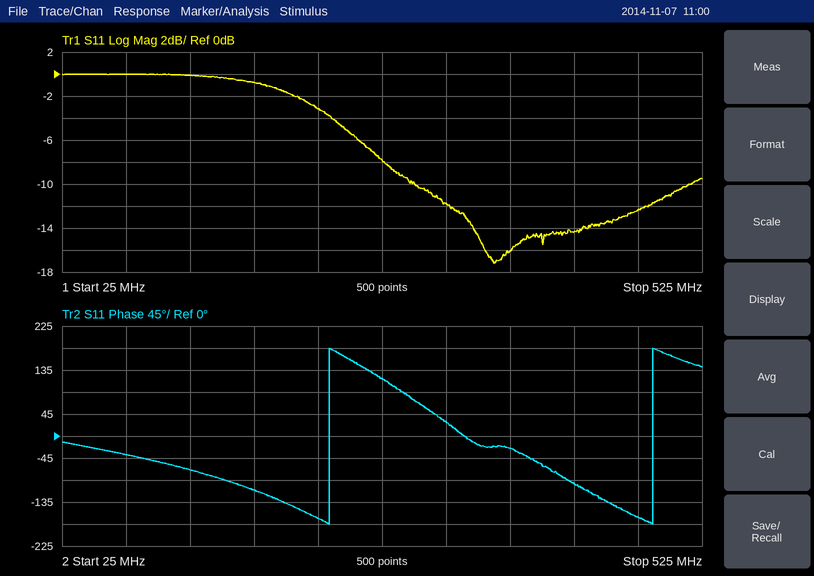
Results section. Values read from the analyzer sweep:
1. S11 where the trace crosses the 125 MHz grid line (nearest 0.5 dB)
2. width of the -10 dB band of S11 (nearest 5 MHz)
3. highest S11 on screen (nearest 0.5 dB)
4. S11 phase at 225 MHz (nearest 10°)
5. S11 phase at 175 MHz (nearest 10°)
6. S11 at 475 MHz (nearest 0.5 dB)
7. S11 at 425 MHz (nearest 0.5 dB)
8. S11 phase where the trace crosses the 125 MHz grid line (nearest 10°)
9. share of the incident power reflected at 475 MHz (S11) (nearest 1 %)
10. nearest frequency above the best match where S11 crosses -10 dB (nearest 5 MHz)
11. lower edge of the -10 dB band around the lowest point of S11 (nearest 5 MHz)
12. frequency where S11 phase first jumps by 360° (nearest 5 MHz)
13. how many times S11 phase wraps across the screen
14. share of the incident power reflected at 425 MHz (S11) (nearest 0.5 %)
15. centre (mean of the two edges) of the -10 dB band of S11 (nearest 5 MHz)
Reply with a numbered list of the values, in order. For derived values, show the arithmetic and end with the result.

1. 0.0 dB
2. 515 MHz − 300 MHz = 215 MHz
3. 0.0 dB
4. -170°
5. -110°
6. -12.5 dB
7. -14.5 dB
8. -70°
9. 10^(-12.5/10) ≈ 6 %
10. 515 MHz
11. 300 MHz
12. 235 MHz
13. 2
14. 10^(-14.5/10) ≈ 3.5 %
15. 410 MHz
